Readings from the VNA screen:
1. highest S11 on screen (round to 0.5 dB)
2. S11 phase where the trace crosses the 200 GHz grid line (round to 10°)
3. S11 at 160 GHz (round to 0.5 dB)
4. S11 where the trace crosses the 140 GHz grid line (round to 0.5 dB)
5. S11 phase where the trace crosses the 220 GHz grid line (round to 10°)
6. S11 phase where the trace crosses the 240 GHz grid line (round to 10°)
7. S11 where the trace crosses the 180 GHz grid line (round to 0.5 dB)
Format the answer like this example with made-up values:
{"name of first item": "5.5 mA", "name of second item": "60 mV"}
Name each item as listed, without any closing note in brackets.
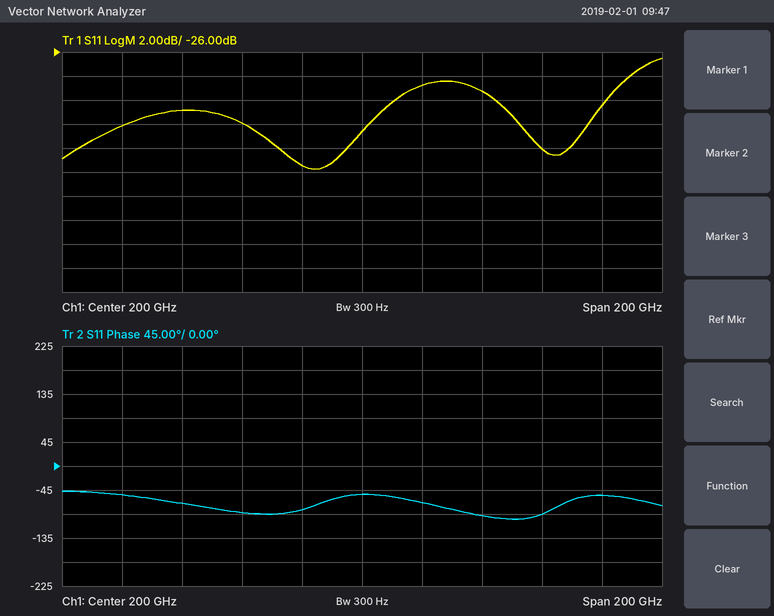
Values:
{"highest S11 on screen": "-26.5 dB", "S11 phase where the trace crosses the 200 GHz grid line": "-50°", "S11 at 160 GHz": "-32.0 dB", "S11 where the trace crosses the 140 GHz grid line": "-31.0 dB", "S11 phase where the trace crosses the 220 GHz grid line": "-70°", "S11 phase where the trace crosses the 240 GHz grid line": "-90°", "S11 where the trace crosses the 180 GHz grid line": "-35.5 dB"}
